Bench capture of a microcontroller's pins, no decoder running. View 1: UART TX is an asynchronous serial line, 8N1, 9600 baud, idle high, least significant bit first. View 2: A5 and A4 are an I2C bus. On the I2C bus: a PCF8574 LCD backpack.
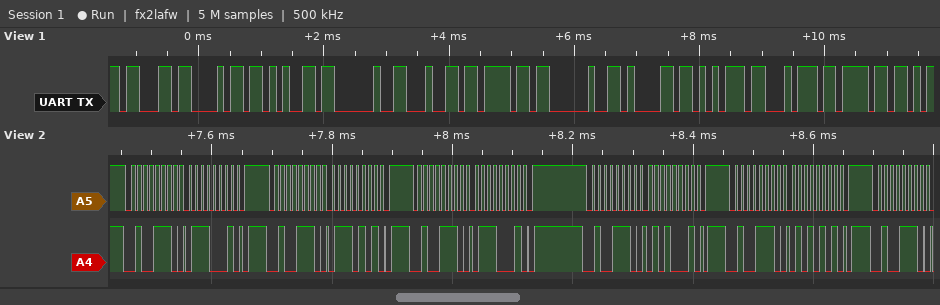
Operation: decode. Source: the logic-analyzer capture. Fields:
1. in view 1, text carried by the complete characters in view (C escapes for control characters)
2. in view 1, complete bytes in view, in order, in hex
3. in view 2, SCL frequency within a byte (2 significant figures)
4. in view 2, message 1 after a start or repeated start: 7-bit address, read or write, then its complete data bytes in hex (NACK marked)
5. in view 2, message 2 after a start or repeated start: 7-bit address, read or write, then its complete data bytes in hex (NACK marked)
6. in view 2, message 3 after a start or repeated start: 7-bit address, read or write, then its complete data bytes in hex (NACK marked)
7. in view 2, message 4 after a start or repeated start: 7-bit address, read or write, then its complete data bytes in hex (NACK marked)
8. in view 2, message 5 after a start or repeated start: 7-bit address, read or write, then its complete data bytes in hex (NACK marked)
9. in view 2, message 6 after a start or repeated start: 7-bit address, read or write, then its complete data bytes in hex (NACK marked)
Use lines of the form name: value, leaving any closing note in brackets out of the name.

in view 1, text carried by the complete characters in view: "che do auto"
in view 1, complete bytes in view, in order, in hex: 63 68 65 20 64 6F 20 61 75 74 6F
in view 2, SCL frequency within a byte: 100 kHz
in view 2, message 1 after a start or repeated start: 7-bit address, read or write, then its complete data bytes in hex: 0x27 write: 71
in view 2, message 2 after a start or repeated start: 7-bit address, read or write, then its complete data bytes in hex: 0x27 write: 75
in view 2, message 3 after a start or repeated start: 7-bit address, read or write, then its complete data bytes in hex: 0x27 write: 71
in view 2, message 4 after a start or repeated start: 7-bit address, read or write, then its complete data bytes in hex: 0x27 write: 51
in view 2, message 5 after a start or repeated start: 7-bit address, read or write, then its complete data bytes in hex: 0x27 write: 55
in view 2, message 6 after a start or repeated start: 7-bit address, read or write, then its complete data bytes in hex: 0x27 write
